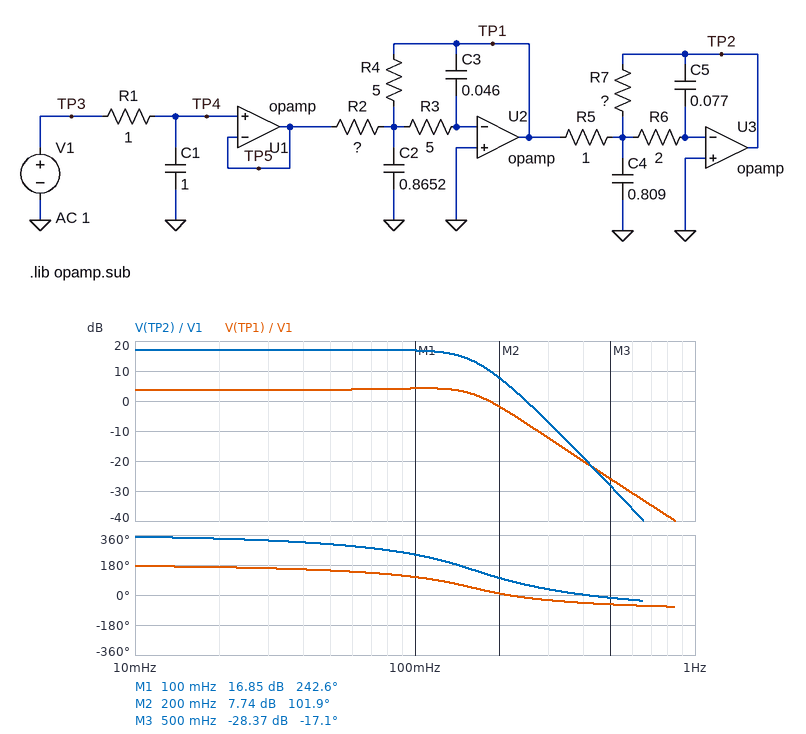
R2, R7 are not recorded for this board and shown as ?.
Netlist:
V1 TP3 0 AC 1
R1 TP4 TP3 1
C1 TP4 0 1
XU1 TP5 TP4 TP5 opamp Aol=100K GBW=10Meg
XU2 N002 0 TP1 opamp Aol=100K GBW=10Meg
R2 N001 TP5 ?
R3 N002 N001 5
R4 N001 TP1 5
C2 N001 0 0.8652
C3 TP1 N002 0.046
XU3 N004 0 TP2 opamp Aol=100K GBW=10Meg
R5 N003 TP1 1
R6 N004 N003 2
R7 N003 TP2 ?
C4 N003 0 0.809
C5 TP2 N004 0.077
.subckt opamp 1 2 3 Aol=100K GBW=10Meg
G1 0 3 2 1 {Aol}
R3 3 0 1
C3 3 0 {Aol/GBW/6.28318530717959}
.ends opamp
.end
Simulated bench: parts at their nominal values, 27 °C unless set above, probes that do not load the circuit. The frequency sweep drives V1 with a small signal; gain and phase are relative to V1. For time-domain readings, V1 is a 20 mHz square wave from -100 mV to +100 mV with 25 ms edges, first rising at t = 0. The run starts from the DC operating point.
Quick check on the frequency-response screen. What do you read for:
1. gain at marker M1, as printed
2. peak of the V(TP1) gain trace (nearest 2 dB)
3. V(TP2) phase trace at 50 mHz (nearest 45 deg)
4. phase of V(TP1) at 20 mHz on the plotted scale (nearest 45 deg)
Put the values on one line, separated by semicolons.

16.85 dB; 4 dB; 315 deg; 180 deg
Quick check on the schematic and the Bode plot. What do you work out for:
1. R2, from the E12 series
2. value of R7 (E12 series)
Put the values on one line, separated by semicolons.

3.3 Ω; 4.7 Ω
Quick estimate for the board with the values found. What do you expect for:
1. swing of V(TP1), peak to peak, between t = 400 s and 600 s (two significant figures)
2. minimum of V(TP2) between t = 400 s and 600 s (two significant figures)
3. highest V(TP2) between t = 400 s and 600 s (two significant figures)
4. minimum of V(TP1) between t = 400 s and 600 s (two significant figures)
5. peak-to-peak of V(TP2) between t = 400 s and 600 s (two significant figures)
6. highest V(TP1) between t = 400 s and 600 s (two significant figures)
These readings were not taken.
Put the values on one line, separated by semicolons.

390 mV; -870 mV; 870 mV; -190 mV; 1.7 V; 190 mV
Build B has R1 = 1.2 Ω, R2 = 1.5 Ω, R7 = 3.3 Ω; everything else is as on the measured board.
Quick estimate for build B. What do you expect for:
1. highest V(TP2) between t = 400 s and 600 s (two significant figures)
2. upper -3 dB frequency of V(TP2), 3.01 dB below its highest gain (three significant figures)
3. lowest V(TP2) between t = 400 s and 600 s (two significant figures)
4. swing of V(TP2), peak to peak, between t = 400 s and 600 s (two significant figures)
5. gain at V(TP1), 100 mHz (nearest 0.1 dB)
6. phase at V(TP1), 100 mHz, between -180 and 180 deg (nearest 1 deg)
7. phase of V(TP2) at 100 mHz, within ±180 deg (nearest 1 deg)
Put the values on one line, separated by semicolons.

1.2 V; 119 mHz; -1.2 V; 2.3 V; 8.7 dB; 91 deg; -123 deg
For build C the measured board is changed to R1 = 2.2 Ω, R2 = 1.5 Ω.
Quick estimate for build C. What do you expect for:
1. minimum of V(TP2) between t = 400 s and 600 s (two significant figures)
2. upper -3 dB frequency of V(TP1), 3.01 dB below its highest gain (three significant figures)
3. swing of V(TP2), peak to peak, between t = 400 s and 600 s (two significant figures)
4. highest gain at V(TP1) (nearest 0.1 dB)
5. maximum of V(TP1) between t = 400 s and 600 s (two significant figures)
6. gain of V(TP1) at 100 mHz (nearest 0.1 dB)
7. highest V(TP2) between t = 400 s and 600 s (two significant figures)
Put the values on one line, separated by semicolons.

-1.6 V; 76.8 mHz; 3.1 V; 10.5 dB; 330 mV; 6.0 dB; 1.6 V
